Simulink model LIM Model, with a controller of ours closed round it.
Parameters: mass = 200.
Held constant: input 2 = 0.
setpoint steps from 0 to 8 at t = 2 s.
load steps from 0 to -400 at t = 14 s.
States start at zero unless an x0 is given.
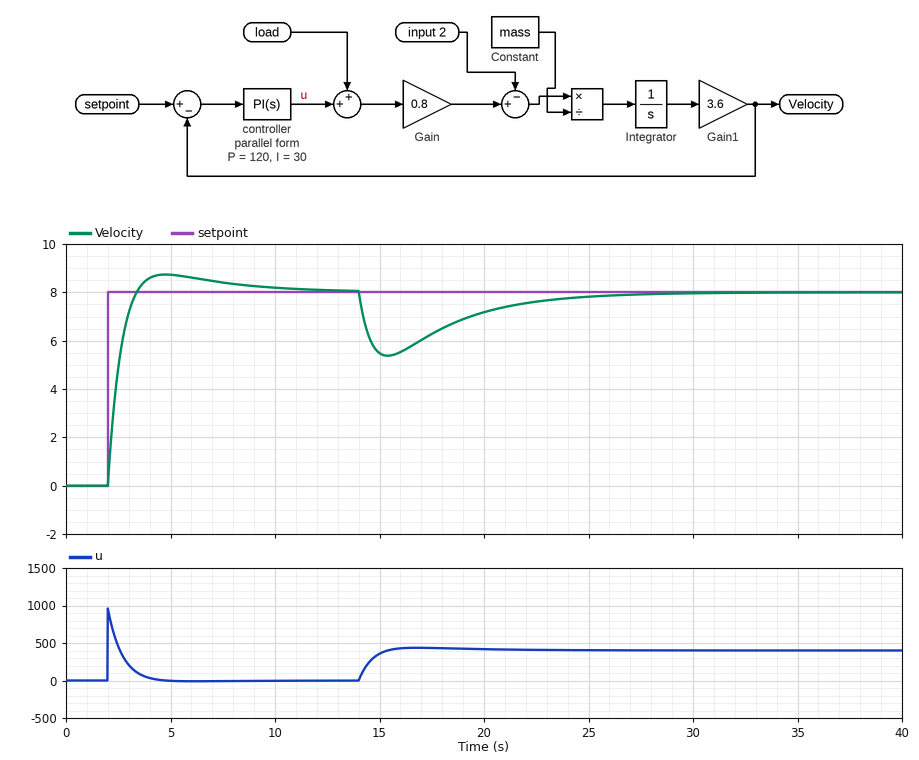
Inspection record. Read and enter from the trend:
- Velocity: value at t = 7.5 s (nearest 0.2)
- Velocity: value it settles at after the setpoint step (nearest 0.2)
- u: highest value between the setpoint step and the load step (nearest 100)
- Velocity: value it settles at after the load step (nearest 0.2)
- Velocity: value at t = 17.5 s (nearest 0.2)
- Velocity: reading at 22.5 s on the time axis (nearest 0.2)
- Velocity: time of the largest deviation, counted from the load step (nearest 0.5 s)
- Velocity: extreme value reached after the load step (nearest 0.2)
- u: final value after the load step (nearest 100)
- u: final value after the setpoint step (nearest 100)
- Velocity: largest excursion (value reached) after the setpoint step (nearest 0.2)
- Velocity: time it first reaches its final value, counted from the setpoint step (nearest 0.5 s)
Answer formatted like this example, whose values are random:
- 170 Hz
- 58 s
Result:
- 8.4
- 8.0
- 1000
- 8.0
- 6.2
- 7.6
- 1.5 s
- 5.4
- 400
- 0
- 8.8
- 1.5 s
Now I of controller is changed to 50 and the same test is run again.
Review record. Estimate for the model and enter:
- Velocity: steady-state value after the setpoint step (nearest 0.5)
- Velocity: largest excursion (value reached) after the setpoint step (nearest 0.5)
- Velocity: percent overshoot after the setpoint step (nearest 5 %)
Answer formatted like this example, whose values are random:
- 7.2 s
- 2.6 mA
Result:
- 8.0
- 9.0
- 15 %
